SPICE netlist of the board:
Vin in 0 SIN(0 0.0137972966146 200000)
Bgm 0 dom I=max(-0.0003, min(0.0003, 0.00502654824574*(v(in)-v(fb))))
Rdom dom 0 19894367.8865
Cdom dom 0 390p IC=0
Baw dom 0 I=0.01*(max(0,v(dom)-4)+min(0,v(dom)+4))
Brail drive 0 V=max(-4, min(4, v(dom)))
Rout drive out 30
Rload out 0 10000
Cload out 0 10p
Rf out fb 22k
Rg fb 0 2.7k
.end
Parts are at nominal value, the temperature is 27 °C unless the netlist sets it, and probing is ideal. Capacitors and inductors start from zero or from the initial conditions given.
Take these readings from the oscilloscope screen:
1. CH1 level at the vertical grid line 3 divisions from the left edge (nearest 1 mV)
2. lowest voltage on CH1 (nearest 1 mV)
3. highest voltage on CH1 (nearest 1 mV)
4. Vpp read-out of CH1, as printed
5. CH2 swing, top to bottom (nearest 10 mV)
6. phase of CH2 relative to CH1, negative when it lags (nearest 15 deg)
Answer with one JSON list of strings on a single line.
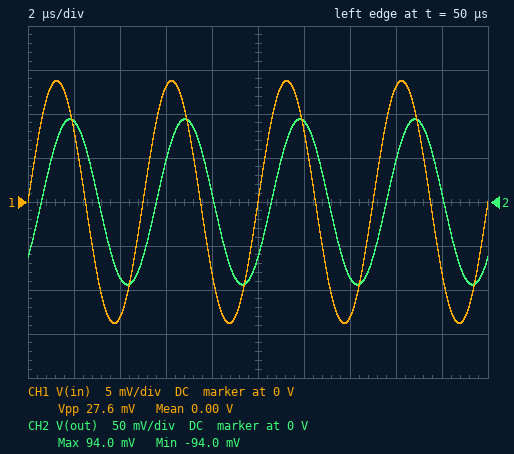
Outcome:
["13 mV", "-14 mV", "14 mV", "27.6 mV", "190 mV", "-45 deg"]
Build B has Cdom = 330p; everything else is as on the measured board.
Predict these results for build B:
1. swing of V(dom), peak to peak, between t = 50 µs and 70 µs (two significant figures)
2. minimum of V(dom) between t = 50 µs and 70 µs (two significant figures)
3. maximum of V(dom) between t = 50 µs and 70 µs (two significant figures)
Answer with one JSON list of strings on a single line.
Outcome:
["200 mV", "-100 mV", "100 mV"]
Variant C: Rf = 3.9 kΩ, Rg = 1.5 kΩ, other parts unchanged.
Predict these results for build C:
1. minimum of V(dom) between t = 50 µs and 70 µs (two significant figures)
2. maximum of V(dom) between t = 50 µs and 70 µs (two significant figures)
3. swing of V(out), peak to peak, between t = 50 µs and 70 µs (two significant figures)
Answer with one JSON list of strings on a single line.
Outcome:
["-47 mV", "47 mV", "94 mV"]
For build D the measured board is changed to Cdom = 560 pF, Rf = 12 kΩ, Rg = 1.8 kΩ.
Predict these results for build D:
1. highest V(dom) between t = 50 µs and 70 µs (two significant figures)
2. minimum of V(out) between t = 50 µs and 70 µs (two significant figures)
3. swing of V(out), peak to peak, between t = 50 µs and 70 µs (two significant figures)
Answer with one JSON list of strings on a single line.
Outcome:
["72 mV", "-72 mV", "140 mV"]
